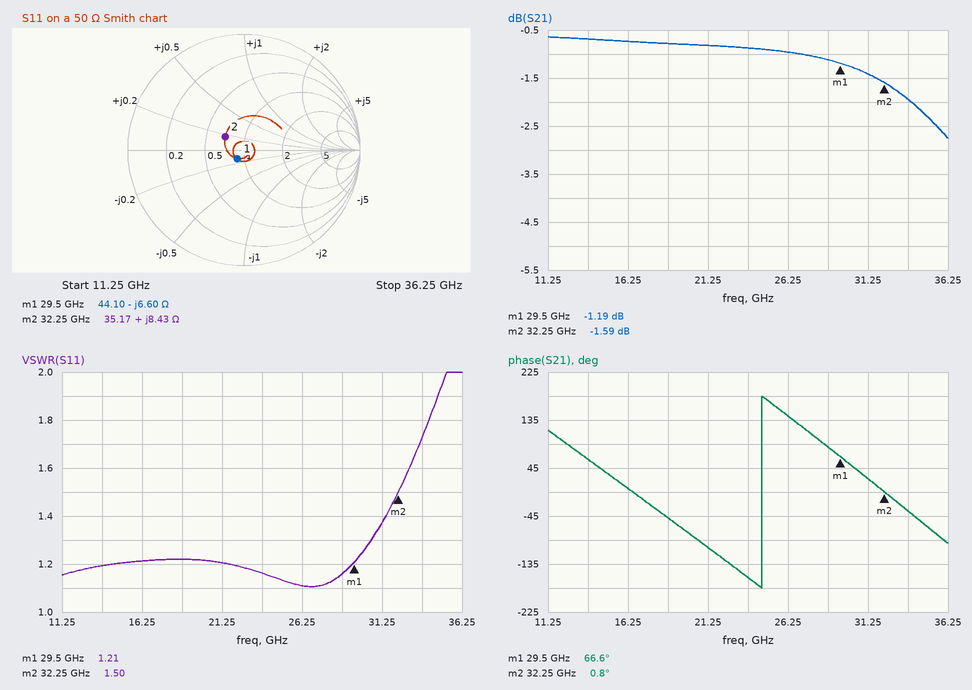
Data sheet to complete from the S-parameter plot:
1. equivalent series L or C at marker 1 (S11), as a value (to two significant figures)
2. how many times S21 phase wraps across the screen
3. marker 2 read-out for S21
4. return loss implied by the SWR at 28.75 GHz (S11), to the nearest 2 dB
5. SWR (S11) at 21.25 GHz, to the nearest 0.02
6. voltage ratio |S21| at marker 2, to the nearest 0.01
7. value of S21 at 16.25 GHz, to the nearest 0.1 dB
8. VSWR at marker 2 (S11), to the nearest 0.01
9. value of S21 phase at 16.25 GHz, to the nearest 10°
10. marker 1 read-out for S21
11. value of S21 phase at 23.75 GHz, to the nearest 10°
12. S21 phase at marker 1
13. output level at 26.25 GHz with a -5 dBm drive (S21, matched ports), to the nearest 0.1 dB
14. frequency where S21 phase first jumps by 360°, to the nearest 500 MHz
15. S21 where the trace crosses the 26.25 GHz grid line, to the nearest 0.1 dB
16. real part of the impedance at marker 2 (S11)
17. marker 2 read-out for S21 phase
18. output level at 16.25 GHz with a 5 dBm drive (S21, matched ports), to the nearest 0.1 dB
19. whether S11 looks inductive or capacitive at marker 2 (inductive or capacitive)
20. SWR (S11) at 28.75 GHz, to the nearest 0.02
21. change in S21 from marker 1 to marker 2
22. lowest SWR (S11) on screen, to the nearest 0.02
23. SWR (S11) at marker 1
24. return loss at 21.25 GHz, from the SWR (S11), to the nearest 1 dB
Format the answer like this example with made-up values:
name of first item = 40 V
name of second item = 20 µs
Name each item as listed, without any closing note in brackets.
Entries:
equivalent series L or C at marker 1 (S11), as a value = 820 fF
how many times S21 phase wraps across the screen = 1
marker 2 read-out for S21 = -1.59 dB
return loss implied by the SWR at 28.75 GHz (S11), to the nearest 2 dB = 22 dB
SWR (S11) at 21.25 GHz, to the nearest 0.02 = 1.20
voltage ratio |S21| at marker 2, to the nearest 0.01 = 0.83
value of S21 at 16.25 GHz, to the nearest 0.1 dB = -0.7 dB
VSWR at marker 2 (S11), to the nearest 0.01 = 1.50
value of S21 phase at 16.25 GHz, to the nearest 10° = 10°
marker 1 read-out for S21 = -1.19 dB
value of S21 phase at 23.75 GHz, to the nearest 10° = -160°
S21 phase at marker 1 = 66.6°
output level at 26.25 GHz with a -5 dBm drive (S21, matched ports), to the nearest 0.1 dB = -6.0 dBm
frequency where S21 phase first jumps by 360°, to the nearest 500 MHz = 24.5 GHz
S21 where the trace crosses the 26.25 GHz grid line, to the nearest 0.1 dB = -1.0 dB
real part of the impedance at marker 2 = 35.17 Ω
marker 2 read-out for S21 phase = 0.8°
output level at 16.25 GHz with a 5 dBm drive (S21, matched ports), to the nearest 0.1 dB = 4.3 dBm
whether S11 looks inductive or capacitive at marker 2 = inductive
SWR (S11) at 28.75 GHz, to the nearest 0.02 = 1.16
change in S21 from marker 1 to marker 2 = -0.40 dB
lowest SWR (S11) on screen, to the nearest 0.02 = 1.10
SWR (S11) at marker 1 = 1.21
return loss at 21.25 GHz, from the SWR (S11), to the nearest 1 dB = 21 dB
